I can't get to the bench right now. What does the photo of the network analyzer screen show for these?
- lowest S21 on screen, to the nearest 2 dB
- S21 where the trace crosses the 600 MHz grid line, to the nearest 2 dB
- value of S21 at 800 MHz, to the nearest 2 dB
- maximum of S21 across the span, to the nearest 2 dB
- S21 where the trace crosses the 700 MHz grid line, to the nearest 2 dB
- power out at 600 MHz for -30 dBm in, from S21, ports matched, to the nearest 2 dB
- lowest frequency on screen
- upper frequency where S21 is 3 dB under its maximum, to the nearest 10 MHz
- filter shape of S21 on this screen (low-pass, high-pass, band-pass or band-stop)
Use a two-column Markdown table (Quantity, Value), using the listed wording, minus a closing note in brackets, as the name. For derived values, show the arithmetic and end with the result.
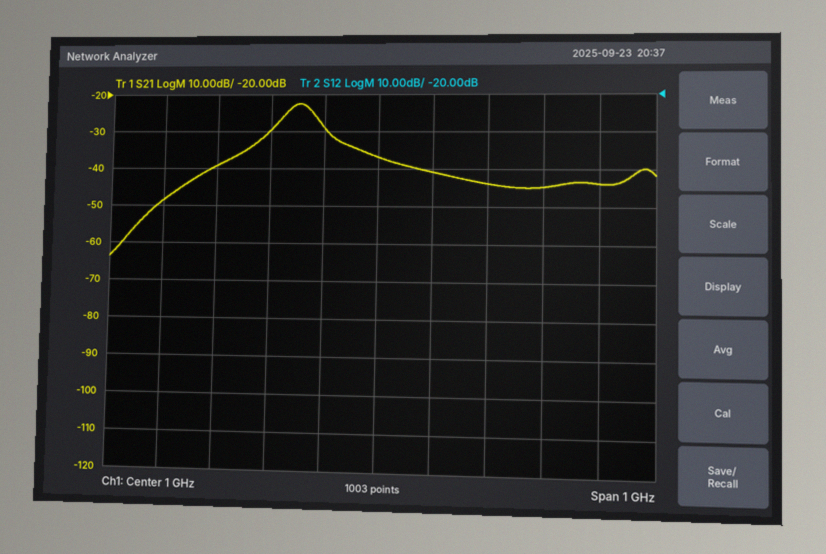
| Quantity | Value |
|---|---|
| lowest S21 on screen, to the nearest 2 dB | -64 dB |
| S21 where the trace crosses the 600 MHz grid line, to the nearest 2 dB | -48 dB |
| value of S21 at 800 MHz, to the nearest 2 dB | -30 dB |
| maximum of S21 across the span, to the nearest 2 dB | -22 dB |
| S21 where the trace crosses the 700 MHz grid line, to the nearest 2 dB | -40 dB |
| power out at 600 MHz for -30 dBm in, from S21, ports matched, to the nearest 2 dB | -30 dBm + (-48 dB) = -78 dBm |
| lowest frequency on screen | 500 MHz |
| upper frequency where S21 is 3 dB under its maximum, to the nearest 10 MHz | 880 MHz |
| filter shape of S21 on this screen | band-pass |
